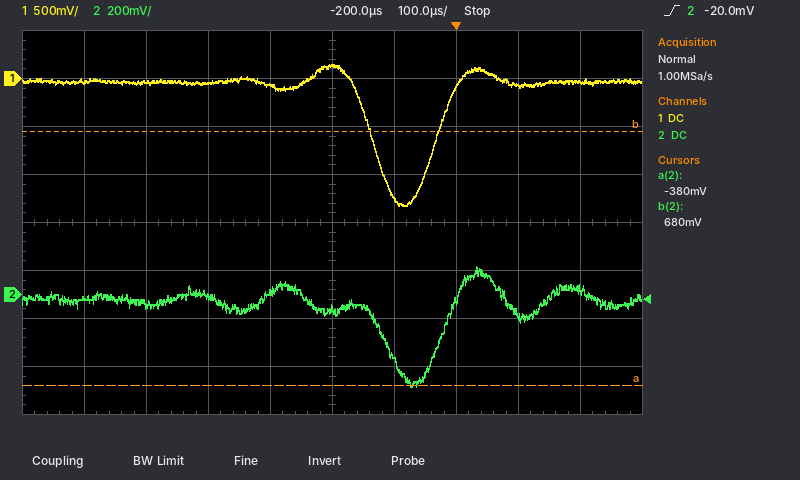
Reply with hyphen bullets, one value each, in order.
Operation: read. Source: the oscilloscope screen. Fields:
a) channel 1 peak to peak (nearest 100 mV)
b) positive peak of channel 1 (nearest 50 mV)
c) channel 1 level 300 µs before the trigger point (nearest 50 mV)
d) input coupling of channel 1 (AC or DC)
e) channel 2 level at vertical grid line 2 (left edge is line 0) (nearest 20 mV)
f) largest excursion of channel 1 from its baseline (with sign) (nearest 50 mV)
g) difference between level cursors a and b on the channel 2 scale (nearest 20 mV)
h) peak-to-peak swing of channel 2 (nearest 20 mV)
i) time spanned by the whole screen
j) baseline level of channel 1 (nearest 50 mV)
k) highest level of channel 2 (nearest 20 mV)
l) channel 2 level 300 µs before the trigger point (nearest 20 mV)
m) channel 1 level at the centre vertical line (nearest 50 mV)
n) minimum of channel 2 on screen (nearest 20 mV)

- 1.50 V
- 150 mV
- -50 mV
- DC
- -40 mV
- -1.30 V
- 1.06 V
- 500 mV
- 1 ms
- -50 mV
- 120 mV
- 20 mV
- 150 mV
- -380 mV
